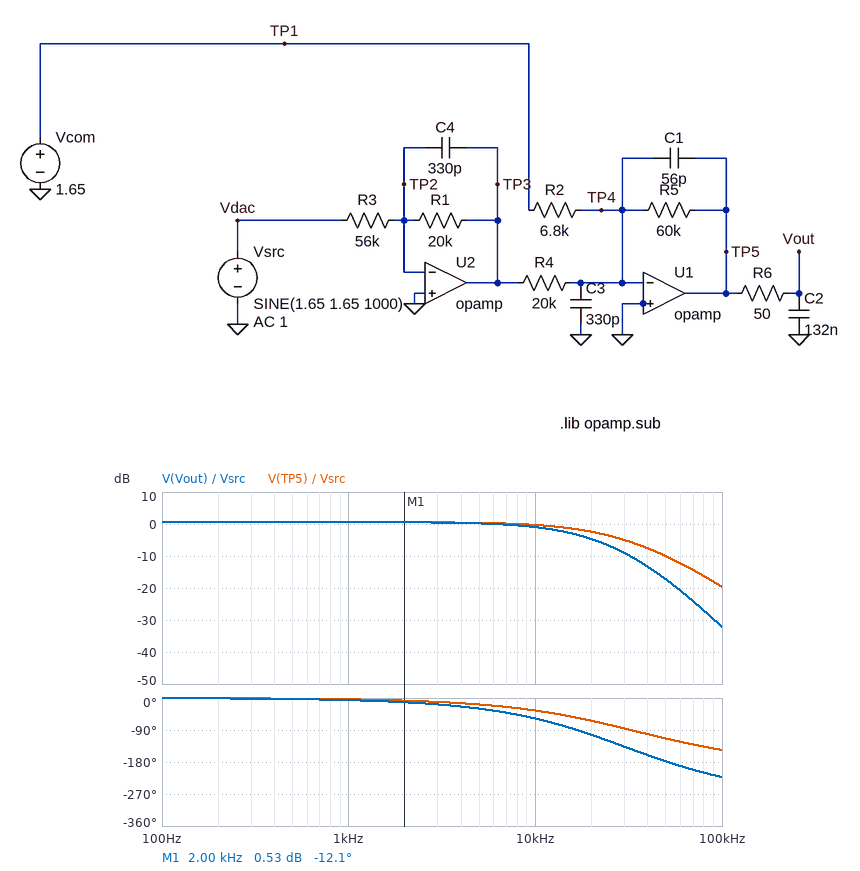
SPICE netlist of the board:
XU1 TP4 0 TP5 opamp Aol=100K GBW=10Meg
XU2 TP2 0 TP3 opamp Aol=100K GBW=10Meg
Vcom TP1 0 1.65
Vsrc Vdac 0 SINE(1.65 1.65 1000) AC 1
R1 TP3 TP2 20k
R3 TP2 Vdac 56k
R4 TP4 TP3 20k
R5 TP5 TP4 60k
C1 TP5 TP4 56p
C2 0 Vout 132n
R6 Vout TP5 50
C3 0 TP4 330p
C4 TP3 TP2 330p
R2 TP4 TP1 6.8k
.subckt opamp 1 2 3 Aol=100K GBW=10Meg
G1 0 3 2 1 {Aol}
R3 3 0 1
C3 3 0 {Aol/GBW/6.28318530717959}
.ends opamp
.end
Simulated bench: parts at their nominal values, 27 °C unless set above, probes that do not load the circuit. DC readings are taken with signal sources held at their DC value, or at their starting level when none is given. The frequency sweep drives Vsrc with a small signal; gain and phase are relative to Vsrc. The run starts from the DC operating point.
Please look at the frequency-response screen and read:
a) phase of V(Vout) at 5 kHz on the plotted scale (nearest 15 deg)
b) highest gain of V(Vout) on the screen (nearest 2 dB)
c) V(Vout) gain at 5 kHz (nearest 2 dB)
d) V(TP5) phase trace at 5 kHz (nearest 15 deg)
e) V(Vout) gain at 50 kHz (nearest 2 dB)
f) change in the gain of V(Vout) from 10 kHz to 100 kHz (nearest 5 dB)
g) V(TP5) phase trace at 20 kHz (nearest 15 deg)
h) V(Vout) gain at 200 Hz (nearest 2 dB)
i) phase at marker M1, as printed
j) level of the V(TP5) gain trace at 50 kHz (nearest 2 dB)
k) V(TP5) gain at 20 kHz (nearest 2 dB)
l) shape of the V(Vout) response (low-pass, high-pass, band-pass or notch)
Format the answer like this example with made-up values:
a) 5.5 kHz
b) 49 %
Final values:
a) -30 deg
b) 0 dB
c) 0 dB
d) -15 deg
e) -18 dB
f) -30 dB
g) -60 deg
h) 0 dB
i) -12.1 deg
j) -10 dB
k) -2 dB
l) low-pass
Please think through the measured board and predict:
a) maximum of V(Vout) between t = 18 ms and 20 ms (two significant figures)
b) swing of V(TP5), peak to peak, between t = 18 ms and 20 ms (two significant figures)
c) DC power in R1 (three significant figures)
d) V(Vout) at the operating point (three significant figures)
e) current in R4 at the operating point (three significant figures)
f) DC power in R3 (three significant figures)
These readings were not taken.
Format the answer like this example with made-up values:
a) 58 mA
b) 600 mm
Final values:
a) -11 V
b) 3.5 V
c) 17.4 µW
d) -12.8 V
e) 29.5 µA
f) 48.6 µW
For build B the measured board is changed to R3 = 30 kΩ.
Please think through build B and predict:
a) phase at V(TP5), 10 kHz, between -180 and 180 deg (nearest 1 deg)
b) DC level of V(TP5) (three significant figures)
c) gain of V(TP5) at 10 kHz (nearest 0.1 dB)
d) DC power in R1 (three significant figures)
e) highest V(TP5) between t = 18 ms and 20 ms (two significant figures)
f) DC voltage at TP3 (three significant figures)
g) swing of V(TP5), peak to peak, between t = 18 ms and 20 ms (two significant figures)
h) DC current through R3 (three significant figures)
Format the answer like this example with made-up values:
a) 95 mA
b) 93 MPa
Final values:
a) -35 deg
b) -11.3 V
c) 5.1 dB
d) 60.5 µW
e) -8.0 V
f) -1.10 V
g) 6.6 V
h) 55.0 µA
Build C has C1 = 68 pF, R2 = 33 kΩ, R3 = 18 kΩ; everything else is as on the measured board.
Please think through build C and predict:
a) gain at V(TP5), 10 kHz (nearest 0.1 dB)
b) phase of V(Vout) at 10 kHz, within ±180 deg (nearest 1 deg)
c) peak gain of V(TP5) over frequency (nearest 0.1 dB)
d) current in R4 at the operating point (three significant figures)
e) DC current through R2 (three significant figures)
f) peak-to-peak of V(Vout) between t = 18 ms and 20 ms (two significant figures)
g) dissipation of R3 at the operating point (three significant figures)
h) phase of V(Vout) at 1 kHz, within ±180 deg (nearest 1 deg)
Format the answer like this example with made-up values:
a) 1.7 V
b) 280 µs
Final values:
a) 9.5 dB
b) -60 deg
c) 10.5 dB
d) 91.7 µA
e) 50.0 µA
f) 11 V
g) 151 µW
h) -6 deg
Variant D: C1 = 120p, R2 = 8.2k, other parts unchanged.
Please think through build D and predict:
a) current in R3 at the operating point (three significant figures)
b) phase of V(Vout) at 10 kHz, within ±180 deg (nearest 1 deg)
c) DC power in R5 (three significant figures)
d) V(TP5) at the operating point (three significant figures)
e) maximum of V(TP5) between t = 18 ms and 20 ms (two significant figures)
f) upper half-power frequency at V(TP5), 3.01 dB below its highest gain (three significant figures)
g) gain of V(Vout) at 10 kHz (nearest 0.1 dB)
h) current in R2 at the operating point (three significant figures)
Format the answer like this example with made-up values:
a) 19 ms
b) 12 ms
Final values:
a) 29.5 µA
b) -70 deg
c) 1.77 mW
d) -10.3 V
e) -8.5 V
f) 14.7 kHz
g) -1.6 dB
h) 201 µA
